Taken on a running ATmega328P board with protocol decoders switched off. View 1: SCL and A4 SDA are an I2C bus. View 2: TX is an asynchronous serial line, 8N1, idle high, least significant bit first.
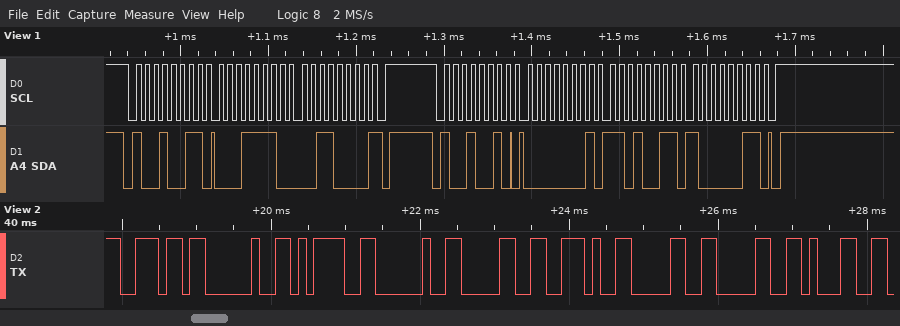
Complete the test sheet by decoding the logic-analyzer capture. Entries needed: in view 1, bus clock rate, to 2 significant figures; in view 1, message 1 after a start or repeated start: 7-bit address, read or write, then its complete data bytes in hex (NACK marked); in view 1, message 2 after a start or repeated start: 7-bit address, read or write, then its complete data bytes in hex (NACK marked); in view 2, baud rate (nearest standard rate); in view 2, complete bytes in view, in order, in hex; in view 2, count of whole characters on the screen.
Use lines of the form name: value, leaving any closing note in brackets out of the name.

in view 1, bus clock rate, to 2 significant figures: 100 kHz
in view 1, message 1 after a start or repeated start: 7-bit address, read or write, then its complete data bytes in hex: 0x49 read: 1E 30 NACK
in view 1, message 2 after a start or repeated start: 7-bit address, read or write, then its complete data bytes in hex: 0x49 write: 01 D3 83
in view 2, baud rate: 9600 baud
in view 2, complete bytes in view, in order, in hex: 6E 20 3D 20 30 2E 30 30 31
in view 2, count of whole characters on the screen: 9
